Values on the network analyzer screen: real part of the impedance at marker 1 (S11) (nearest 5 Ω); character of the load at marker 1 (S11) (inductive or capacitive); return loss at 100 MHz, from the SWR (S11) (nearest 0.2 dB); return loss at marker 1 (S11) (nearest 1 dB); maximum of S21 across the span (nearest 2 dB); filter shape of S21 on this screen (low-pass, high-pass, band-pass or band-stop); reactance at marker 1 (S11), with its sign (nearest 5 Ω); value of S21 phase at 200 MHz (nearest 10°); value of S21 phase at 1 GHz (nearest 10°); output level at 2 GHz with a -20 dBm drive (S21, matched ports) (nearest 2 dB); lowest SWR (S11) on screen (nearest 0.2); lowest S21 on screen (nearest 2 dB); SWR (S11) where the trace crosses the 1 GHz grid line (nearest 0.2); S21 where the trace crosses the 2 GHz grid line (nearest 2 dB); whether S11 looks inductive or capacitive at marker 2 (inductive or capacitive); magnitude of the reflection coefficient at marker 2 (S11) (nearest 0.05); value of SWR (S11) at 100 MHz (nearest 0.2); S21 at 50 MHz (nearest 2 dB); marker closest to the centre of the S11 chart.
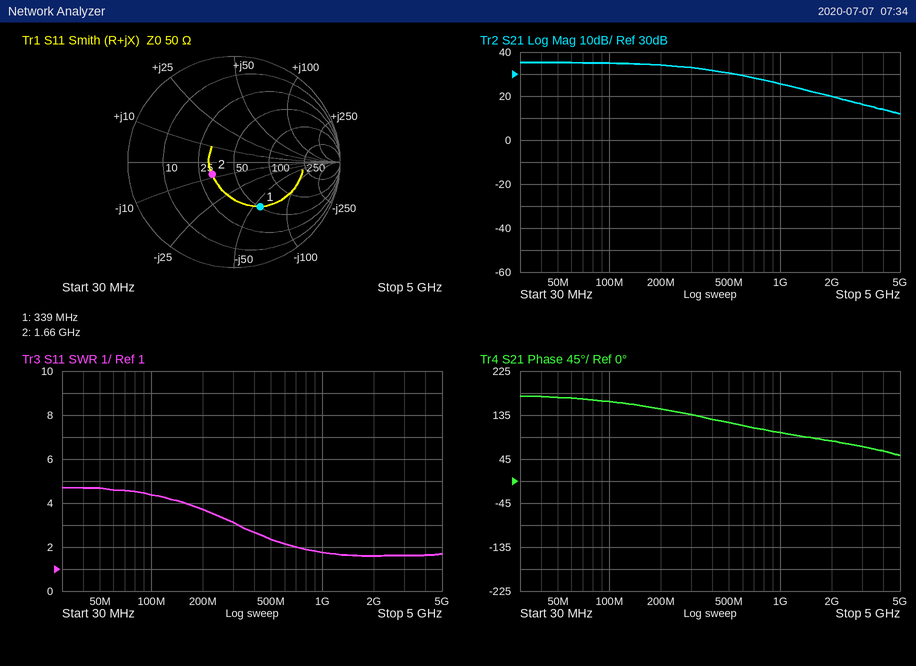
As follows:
50 Ω
capacitive
4.0 dB
6 dB
36 dB
low-pass
-55 Ω
150°
100°
0 dBm
1.6
12 dB
1.8
20 dB
capacitive
0.25
4.4
36 dB
marker 2
